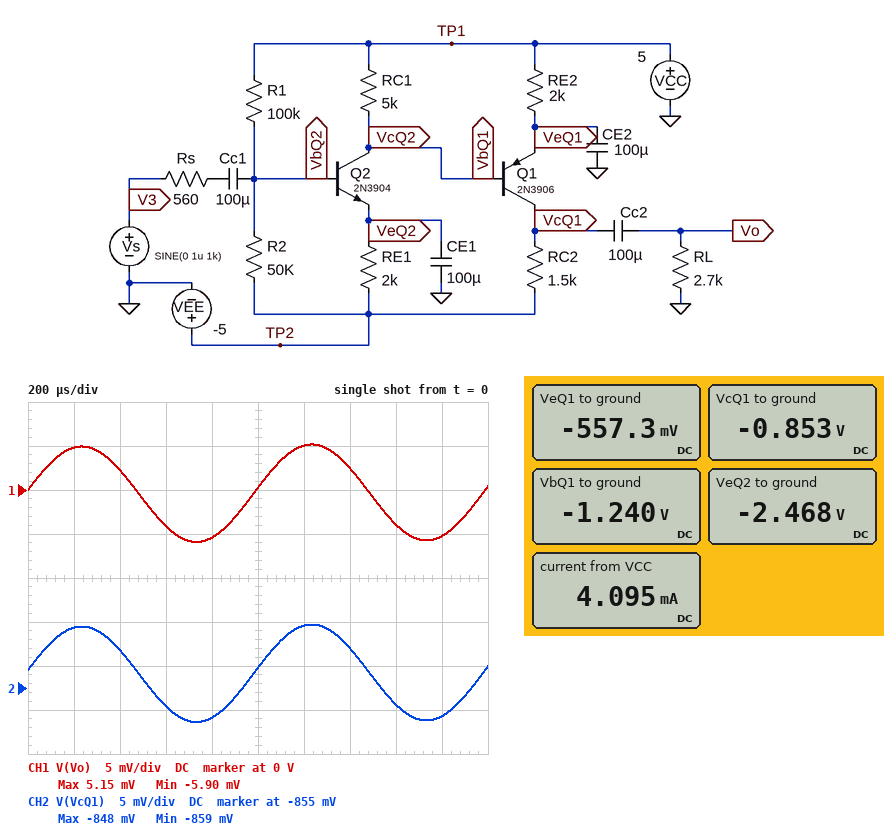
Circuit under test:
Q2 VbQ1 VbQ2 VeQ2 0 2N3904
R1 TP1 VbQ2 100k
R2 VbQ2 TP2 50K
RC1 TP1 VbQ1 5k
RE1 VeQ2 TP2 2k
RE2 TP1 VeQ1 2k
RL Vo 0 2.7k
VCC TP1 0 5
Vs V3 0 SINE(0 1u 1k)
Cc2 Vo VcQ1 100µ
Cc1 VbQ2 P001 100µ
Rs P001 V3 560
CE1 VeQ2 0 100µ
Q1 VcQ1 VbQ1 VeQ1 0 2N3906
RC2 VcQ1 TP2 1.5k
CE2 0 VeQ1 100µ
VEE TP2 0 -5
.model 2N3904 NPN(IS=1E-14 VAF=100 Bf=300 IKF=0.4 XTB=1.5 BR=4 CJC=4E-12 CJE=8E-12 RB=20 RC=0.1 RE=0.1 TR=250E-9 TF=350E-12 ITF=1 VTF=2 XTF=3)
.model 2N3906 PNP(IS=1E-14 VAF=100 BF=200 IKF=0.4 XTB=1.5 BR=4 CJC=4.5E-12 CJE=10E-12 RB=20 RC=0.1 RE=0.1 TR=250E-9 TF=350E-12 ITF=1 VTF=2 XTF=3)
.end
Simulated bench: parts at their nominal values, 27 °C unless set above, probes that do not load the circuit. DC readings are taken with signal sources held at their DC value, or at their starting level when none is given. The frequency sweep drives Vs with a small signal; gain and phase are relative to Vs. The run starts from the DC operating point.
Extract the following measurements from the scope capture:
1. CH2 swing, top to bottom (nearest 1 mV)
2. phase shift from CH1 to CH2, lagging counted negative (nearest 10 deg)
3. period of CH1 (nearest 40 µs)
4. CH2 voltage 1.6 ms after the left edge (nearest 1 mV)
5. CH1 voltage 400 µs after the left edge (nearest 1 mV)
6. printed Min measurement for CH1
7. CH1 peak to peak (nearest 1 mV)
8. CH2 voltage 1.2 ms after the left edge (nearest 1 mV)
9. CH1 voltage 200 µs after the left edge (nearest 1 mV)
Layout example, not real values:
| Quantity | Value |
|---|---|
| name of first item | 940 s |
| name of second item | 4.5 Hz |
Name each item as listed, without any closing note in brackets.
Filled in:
| Quantity | Value |
|---|---|
| CH2 swing, top to bottom | 11 mV |
| phase shift from CH1 to CH2, lagging counted negative | 0 deg |
| period of CH1 | 1.00 ms |
| CH2 voltage 1.6 ms after the left edge | -857 mV |
| CH1 voltage 400 µs after the left edge | 2 mV |
| printed Min measurement for CH1 | -5.90 mV |
| CH1 peak to peak | 11 mV |
| CH2 voltage 1.2 ms after the left edge | -848 mV |
| CH1 voltage 200 µs after the left edge | 5 mV |
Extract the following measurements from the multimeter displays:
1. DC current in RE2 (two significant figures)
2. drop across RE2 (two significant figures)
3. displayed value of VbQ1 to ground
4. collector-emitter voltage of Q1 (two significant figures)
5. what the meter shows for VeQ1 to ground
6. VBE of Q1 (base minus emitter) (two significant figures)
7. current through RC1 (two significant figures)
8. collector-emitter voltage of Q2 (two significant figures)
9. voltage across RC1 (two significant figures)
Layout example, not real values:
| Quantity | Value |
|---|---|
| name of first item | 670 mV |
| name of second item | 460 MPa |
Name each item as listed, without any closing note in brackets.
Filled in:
| Quantity | Value |
|---|---|
| DC current in RE2 | 2.8 mA |
| drop across RE2 | 5.6 V |
| displayed value of VbQ1 to ground | -1.240 V |
| collector-emitter voltage of Q1 | -300 mV |
| what the meter shows for VeQ1 to ground | -557.3 mV |
| VBE of Q1 (base minus emitter) | -680 mV |
| current through RC1 | 1.2 mA |
| collector-emitter voltage of Q2 | 1.2 V |
| voltage across RC1 | 6.2 V |
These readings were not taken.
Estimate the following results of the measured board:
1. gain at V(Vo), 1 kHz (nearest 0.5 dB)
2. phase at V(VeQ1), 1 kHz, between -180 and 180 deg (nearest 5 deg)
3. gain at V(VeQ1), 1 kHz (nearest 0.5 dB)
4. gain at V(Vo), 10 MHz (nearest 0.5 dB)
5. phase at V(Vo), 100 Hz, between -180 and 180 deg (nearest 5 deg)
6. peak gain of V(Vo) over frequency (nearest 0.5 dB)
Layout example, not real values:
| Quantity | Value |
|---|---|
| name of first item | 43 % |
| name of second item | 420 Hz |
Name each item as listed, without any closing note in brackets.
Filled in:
| Quantity | Value |
|---|---|
| gain at V(Vo), 1 kHz | 75.0 dB |
| phase at V(VeQ1), 1 kHz, between -180 and 180 deg | 95 deg |
| gain at V(VeQ1), 1 kHz | 19.0 dB |
| gain at V(Vo), 10 MHz | 36.0 dB |
| phase at V(Vo), 100 Hz, between -180 and 180 deg | 60 deg |
| peak gain of V(Vo) over frequency | 75.0 dB |
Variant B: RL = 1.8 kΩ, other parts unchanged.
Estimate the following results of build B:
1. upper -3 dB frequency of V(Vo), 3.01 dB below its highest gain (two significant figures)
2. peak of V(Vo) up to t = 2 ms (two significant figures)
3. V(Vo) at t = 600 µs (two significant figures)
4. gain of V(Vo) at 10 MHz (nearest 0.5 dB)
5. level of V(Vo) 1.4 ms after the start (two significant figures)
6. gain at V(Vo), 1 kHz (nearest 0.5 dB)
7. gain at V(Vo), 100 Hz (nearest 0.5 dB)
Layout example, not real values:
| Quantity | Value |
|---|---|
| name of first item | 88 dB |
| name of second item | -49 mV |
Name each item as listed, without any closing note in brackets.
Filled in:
| Quantity | Value |
|---|---|
| upper -3 dB frequency of V(Vo), 3.01 dB below its highest gain | 190 kHz |
| peak of V(Vo) up to t = 2 ms | 4.4 mV |
| V(Vo) at t = 600 µs | -3.5 mV |
| gain of V(Vo) at 10 MHz | 35.5 dB |
| level of V(Vo) 1.4 ms after the start | 2.1 mV |
| gain at V(Vo), 1 kHz | 73.5 dB |
| gain at V(Vo), 100 Hz | 71.0 dB |
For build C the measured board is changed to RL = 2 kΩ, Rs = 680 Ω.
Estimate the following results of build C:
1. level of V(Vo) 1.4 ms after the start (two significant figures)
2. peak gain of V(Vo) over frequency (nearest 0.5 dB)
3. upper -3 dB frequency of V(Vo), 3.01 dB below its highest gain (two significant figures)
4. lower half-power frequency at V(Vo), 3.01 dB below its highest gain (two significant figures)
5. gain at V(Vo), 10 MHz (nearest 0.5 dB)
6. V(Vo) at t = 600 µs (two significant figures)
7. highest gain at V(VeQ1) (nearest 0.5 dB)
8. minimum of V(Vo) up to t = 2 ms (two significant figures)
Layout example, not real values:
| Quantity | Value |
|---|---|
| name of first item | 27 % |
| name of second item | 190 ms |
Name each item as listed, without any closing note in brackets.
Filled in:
| Quantity | Value |
|---|---|
| level of V(Vo) 1.4 ms after the start | 2.2 mV |
| peak gain of V(Vo) over frequency | 73.5 dB |
| upper -3 dB frequency of V(Vo), 3.01 dB below its highest gain | 180 kHz |
| lower half-power frequency at V(Vo), 3.01 dB below its highest gain | 91 Hz |
| gain at V(Vo), 10 MHz | 34.5 dB |
| V(Vo) at t = 600 µs | -3.6 mV |
| highest gain at V(VeQ1) | 38.0 dB |
| minimum of V(Vo) up to t = 2 ms | -5.2 mV |
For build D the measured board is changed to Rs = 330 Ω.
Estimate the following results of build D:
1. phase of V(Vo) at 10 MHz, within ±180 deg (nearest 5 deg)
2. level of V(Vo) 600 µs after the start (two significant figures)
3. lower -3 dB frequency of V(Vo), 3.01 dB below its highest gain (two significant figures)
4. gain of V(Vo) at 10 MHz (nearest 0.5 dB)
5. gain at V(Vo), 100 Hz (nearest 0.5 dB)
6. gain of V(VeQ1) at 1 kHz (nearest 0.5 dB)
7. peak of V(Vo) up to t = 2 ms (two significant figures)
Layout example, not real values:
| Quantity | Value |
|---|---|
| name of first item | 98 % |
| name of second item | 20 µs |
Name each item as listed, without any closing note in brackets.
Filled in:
| Quantity | Value |
|---|---|
| phase of V(Vo) at 10 MHz, within ±180 deg | -125 deg |
| level of V(Vo) 600 µs after the start | -4.3 mV |
| lower -3 dB frequency of V(Vo), 3.01 dB below its highest gain | 94 Hz |
| gain of V(Vo) at 10 MHz | 38.0 dB |
| gain at V(Vo), 100 Hz | 72.5 dB |
| gain of V(VeQ1) at 1 kHz | 19.5 dB |
| peak of V(Vo) up to t = 2 ms | 5.4 mV |
